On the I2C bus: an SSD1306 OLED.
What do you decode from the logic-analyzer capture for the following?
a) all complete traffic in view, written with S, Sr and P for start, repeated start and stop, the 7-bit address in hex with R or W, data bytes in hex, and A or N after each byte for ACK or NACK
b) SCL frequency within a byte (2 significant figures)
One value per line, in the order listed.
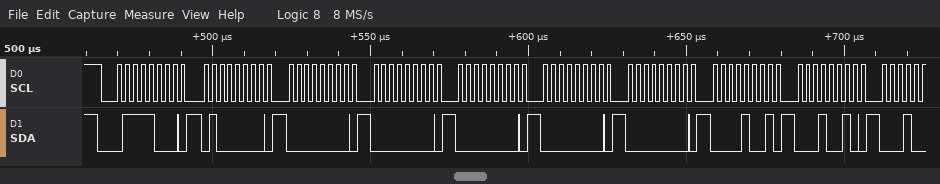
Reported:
S 3CW A 40 A 00 A 00 A 00 A 00 A 00 A 09 A 12 A
400 kHz
